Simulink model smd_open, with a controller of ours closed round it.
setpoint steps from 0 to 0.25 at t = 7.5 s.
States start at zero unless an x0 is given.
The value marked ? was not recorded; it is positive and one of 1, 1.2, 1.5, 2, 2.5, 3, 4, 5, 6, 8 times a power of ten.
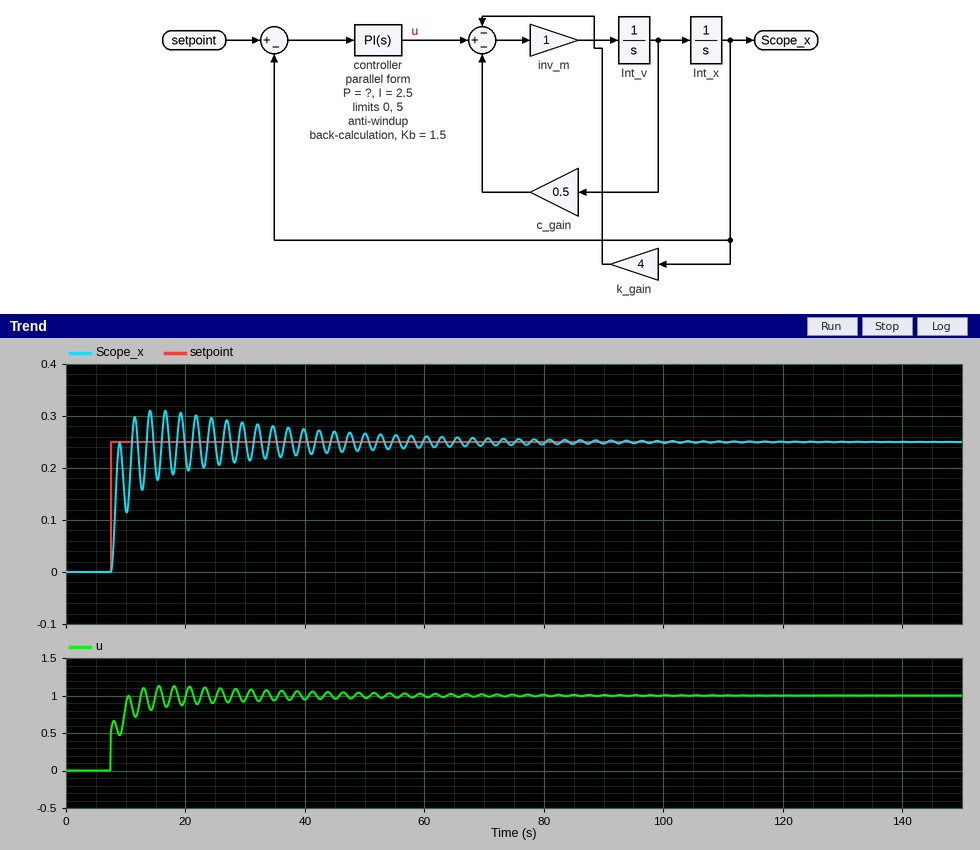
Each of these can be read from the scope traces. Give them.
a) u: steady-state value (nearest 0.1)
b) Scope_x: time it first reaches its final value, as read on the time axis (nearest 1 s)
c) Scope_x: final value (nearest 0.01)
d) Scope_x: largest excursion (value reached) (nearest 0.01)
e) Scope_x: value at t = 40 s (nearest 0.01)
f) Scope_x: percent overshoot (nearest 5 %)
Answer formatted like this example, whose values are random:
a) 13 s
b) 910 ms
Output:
a) 1.0
b) 11 s
c) 0.25
d) 0.31
e) 0.27
f) 25 %
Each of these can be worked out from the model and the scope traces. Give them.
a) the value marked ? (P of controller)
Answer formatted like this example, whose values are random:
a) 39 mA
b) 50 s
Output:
a) 2
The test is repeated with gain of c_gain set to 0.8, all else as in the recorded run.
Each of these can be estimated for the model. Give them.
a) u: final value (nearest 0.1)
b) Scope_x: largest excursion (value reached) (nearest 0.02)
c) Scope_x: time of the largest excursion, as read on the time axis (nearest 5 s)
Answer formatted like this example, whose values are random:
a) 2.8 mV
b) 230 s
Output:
a) 1.0
b) 0.26
c) 15 s
